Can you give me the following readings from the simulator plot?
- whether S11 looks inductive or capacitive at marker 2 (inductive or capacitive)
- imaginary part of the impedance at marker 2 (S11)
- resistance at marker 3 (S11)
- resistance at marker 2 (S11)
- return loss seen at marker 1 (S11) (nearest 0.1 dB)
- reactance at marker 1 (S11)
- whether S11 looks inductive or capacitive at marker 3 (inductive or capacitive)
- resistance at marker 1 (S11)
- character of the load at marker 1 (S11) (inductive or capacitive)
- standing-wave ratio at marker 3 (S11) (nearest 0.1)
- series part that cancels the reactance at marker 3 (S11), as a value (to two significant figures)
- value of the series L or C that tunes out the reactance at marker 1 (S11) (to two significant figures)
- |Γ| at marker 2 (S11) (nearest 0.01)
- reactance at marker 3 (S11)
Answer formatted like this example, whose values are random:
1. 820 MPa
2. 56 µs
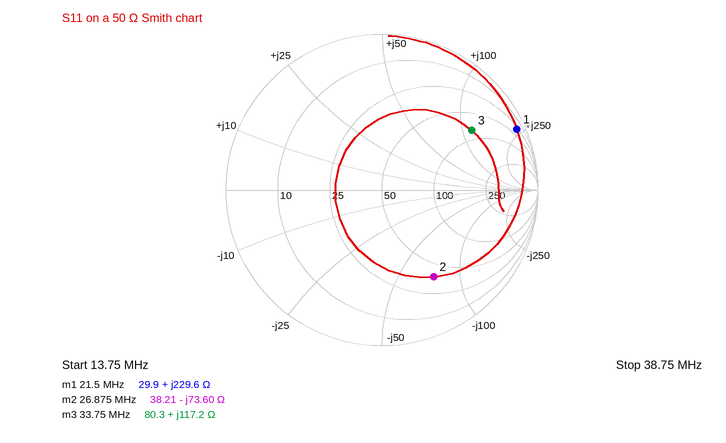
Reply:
1. capacitive
2. -73.60 Ω
3. 80.3 Ω
4. 38.21 Ω
5. 0.5 dB
6. +229.6 Ω
7. inductive
8. 29.9 Ω
9. inductive
10. 5.5
11. 40 pF
12. 32 pF
13. 0.65
14. +117.2 Ω
